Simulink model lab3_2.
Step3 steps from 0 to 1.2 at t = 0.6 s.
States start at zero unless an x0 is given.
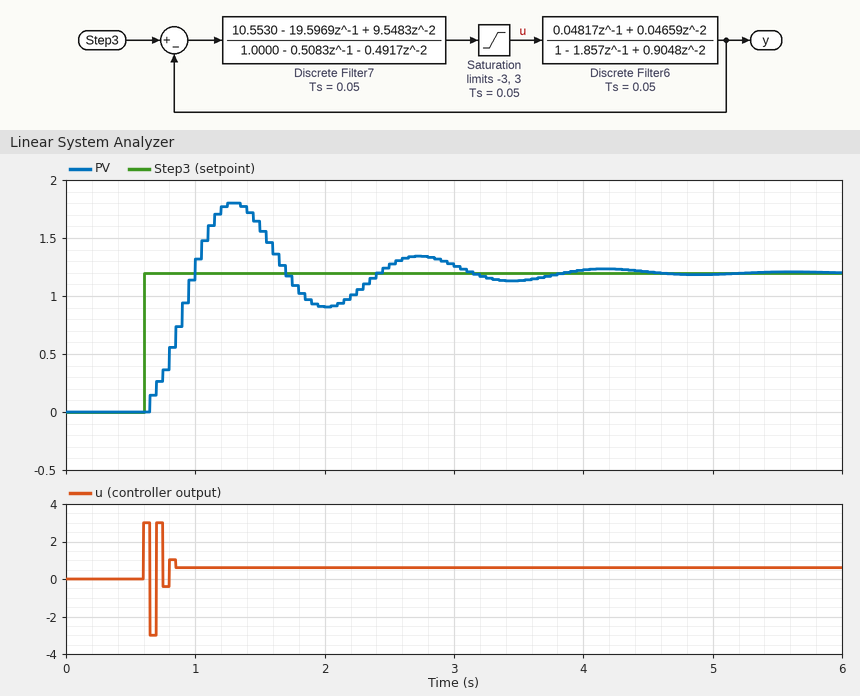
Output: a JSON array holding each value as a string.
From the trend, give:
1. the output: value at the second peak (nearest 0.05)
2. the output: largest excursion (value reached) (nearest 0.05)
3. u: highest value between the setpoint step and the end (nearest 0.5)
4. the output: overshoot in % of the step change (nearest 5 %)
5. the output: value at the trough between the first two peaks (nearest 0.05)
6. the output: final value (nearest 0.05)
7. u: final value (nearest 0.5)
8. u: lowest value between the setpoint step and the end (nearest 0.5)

["1.35", "1.80", "3.0", "50 %", "0.90", "1.20", "0.5", "-3.0"]
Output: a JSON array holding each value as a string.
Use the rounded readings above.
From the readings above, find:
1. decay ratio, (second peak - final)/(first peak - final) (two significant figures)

["0.25"]
